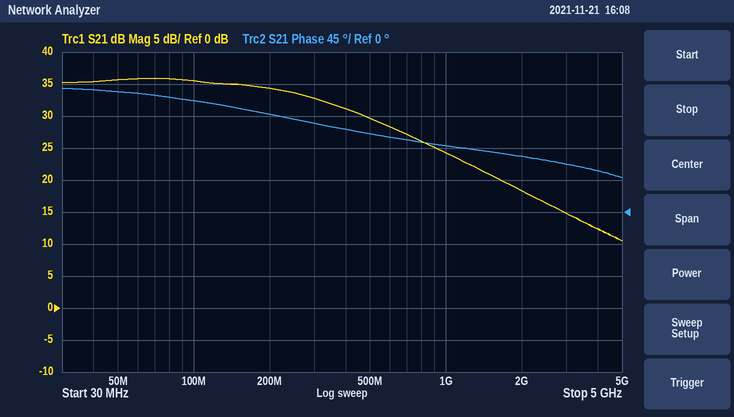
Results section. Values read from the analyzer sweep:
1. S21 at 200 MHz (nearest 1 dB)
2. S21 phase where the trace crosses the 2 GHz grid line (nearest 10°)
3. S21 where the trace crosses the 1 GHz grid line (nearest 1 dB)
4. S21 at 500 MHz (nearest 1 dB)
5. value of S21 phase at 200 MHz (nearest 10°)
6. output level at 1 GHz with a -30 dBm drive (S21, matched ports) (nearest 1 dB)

34 dB
80°
24 dB
30 dB
140°
-6 dBm
